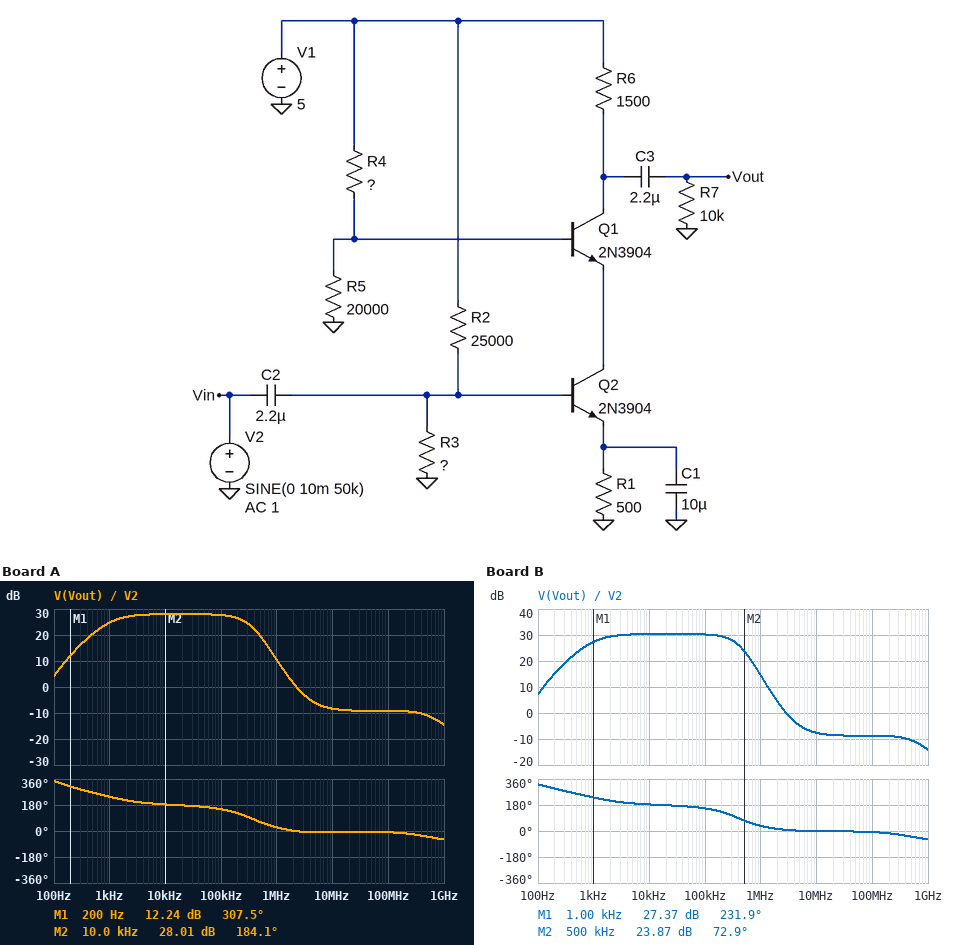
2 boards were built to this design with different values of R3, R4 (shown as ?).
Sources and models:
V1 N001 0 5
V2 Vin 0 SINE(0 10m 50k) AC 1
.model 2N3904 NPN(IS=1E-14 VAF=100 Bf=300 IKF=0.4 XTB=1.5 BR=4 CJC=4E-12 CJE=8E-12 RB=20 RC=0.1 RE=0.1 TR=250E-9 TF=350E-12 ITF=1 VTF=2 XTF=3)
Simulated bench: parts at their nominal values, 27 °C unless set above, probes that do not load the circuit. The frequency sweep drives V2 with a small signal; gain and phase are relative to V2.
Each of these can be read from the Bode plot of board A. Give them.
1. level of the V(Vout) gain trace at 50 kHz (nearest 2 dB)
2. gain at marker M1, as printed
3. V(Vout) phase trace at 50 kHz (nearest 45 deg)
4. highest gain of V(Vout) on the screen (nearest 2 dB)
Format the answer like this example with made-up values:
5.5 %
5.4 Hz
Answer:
28 dB
12.24 dB
180 deg
28 dB
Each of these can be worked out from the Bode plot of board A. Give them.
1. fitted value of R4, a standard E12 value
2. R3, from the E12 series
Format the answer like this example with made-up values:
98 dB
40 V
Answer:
47 kΩ
33 kΩ
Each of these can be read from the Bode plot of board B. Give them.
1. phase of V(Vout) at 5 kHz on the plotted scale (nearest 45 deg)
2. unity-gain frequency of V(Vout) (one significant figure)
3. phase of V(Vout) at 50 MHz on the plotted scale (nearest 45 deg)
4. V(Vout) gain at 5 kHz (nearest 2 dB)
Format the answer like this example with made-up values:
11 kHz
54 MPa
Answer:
180 deg
3 MHz
0 deg
30 dB
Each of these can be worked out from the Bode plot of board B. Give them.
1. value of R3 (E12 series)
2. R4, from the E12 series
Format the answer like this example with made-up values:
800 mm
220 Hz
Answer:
18 kΩ
47 kΩ
